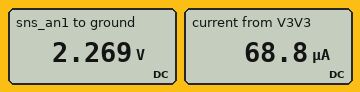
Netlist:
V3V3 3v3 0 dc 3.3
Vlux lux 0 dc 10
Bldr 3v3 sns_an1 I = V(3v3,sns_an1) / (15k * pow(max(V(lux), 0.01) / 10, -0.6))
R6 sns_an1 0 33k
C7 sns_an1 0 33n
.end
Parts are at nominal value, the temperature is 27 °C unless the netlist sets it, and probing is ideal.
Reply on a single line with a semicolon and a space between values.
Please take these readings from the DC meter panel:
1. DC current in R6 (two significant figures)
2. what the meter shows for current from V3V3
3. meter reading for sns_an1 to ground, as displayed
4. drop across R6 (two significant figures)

69 µA; 68.8 µA; 2.269 V; 2.3 V
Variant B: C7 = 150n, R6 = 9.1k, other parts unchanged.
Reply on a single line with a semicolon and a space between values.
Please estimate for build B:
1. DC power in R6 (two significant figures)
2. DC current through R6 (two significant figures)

170 µW; 140 µA
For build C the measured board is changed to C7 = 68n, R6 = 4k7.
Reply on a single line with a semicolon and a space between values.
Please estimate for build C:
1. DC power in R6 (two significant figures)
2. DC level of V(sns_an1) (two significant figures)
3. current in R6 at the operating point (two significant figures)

130 µW; 790 mV; 170 µA
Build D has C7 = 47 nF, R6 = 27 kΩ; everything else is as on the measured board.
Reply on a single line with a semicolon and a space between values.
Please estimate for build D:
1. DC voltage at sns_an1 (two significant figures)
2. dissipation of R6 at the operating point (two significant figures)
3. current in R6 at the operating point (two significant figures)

2.1 V; 170 µW; 79 µA
